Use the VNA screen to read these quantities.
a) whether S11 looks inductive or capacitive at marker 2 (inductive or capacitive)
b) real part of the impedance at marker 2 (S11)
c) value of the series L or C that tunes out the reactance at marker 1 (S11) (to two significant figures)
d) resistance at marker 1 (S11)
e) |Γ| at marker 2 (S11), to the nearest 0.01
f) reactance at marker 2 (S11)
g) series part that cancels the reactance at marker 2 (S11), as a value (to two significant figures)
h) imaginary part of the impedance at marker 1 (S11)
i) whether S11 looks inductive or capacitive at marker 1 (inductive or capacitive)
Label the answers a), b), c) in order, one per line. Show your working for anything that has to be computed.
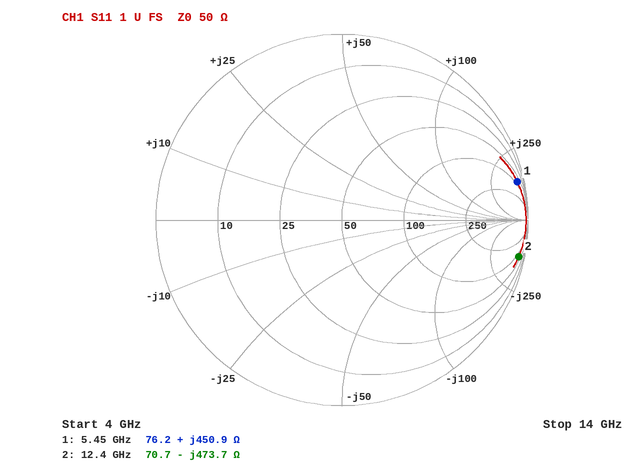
a) capacitive
b) 70.7 Ω
c) C = 1/(2π × 5.45 GHz × 450.9 Ω) ≈ 65 fF
d) 76.2 Ω
e) 0.97
f) -473.7 Ω
g) L = 473.7 Ω/(2π × 12.4 GHz) ≈ 6.1 nH
h) +450.9 Ω
i) inductive
